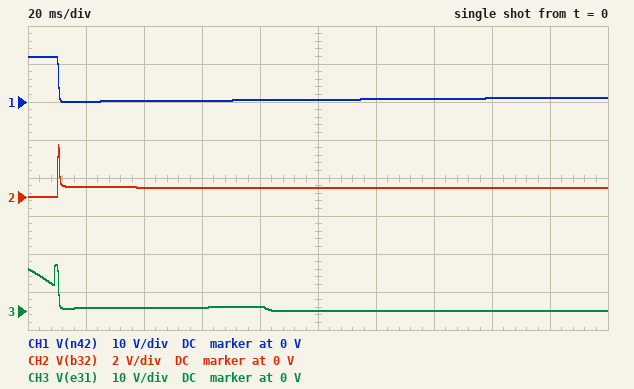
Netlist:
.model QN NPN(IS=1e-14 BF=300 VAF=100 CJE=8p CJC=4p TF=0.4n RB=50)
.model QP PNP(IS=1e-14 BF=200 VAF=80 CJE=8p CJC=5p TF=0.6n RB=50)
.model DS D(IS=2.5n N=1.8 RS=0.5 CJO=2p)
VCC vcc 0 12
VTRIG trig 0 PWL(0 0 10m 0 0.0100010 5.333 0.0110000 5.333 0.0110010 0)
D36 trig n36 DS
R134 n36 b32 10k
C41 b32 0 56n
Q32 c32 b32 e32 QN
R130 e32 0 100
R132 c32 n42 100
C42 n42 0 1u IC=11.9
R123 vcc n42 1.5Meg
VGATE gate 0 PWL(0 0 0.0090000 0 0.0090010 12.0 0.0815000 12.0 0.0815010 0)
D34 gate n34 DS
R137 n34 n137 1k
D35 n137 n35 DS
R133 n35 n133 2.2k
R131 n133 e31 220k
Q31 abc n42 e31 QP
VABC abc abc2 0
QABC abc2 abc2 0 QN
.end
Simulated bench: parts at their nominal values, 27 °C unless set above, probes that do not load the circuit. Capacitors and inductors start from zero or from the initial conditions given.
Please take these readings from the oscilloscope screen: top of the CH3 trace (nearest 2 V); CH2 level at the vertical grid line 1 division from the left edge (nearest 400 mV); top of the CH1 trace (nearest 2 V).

12 V
400 mV
12 V
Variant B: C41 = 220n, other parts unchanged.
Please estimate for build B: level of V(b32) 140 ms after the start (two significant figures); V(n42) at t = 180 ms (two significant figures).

510 mV
740 mV
